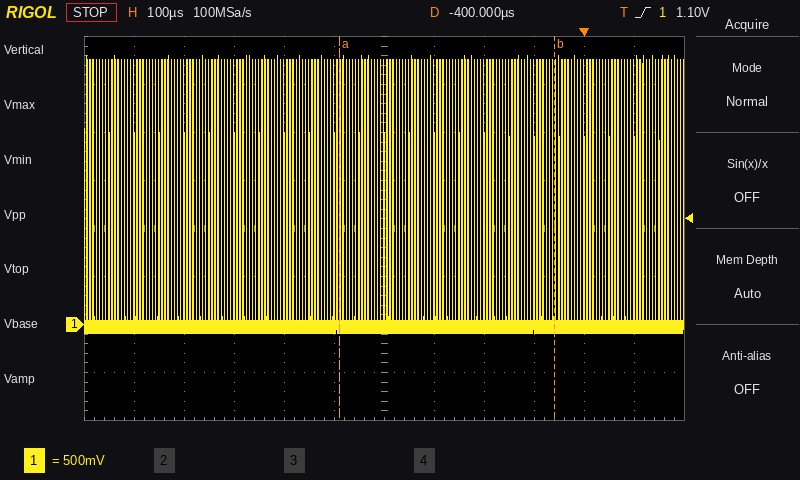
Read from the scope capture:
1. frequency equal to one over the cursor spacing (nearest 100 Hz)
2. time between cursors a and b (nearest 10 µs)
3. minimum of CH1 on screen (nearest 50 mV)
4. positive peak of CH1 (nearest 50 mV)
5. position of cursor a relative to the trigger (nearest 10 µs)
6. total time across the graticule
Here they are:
2.3 kHz
430 µs
-100 mV
2.80 V
-490 µs
1.2 ms
